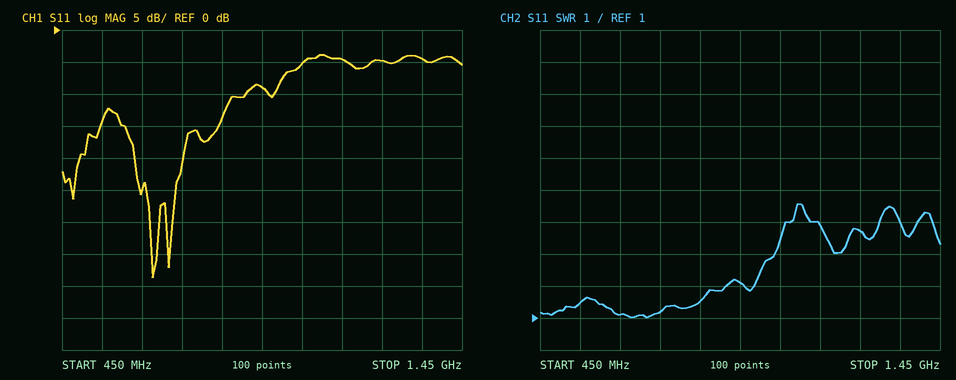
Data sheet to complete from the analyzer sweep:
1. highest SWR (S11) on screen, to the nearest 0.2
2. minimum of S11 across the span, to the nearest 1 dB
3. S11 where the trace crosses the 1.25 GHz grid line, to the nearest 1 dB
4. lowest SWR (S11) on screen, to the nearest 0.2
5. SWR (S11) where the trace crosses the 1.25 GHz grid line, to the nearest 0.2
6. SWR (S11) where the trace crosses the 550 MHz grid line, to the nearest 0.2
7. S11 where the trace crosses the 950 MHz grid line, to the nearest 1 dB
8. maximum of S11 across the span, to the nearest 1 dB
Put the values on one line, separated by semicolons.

4.6; -39 dB; -5 dB; 1.0; 3.8; 1.4; -9 dB; -4 dB
